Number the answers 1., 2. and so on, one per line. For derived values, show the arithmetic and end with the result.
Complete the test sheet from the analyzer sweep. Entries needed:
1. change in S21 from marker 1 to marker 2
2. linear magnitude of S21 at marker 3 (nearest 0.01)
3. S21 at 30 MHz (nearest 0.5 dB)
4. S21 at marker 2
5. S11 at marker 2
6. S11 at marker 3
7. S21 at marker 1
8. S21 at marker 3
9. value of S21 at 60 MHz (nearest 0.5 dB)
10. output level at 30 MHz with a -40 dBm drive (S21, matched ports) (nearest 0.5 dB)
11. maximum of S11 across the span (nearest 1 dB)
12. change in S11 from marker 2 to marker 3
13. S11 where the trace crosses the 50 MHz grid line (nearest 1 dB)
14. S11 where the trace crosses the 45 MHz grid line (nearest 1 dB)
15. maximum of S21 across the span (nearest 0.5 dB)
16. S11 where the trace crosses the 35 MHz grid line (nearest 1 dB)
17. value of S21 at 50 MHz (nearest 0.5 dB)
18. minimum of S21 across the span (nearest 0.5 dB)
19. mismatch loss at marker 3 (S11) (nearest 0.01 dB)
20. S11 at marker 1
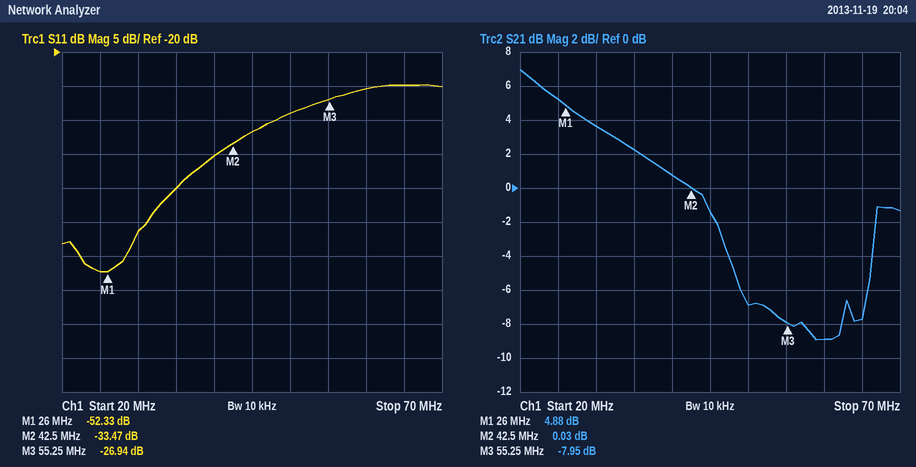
1. 0.03 − (4.88) = -4.85 dB
2. 10^(-7.95/20) ≈ 0.40
3. 3.5 dB
4. 0.03 dB
5. -33.47 dB
6. -26.94 dB
7. 4.88 dB
8. -7.95 dB
9. -9.0 dB
10. -40 dBm + (3.5 dB) = -36.5 dBm
11. -25 dB
12. -26.94 − (-33.47) = 6.53 dB
13. -29 dB
14. -32 dB
15. 7.0 dB
16. -40 dB
17. -7.0 dB
18. -9.0 dB
19. −10 log10(1 − 10^(-26.94/10)) ≈ 0.01 dB
20. -52.33 dB
